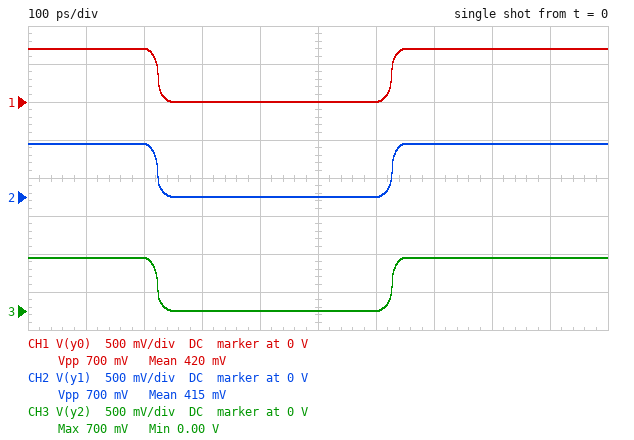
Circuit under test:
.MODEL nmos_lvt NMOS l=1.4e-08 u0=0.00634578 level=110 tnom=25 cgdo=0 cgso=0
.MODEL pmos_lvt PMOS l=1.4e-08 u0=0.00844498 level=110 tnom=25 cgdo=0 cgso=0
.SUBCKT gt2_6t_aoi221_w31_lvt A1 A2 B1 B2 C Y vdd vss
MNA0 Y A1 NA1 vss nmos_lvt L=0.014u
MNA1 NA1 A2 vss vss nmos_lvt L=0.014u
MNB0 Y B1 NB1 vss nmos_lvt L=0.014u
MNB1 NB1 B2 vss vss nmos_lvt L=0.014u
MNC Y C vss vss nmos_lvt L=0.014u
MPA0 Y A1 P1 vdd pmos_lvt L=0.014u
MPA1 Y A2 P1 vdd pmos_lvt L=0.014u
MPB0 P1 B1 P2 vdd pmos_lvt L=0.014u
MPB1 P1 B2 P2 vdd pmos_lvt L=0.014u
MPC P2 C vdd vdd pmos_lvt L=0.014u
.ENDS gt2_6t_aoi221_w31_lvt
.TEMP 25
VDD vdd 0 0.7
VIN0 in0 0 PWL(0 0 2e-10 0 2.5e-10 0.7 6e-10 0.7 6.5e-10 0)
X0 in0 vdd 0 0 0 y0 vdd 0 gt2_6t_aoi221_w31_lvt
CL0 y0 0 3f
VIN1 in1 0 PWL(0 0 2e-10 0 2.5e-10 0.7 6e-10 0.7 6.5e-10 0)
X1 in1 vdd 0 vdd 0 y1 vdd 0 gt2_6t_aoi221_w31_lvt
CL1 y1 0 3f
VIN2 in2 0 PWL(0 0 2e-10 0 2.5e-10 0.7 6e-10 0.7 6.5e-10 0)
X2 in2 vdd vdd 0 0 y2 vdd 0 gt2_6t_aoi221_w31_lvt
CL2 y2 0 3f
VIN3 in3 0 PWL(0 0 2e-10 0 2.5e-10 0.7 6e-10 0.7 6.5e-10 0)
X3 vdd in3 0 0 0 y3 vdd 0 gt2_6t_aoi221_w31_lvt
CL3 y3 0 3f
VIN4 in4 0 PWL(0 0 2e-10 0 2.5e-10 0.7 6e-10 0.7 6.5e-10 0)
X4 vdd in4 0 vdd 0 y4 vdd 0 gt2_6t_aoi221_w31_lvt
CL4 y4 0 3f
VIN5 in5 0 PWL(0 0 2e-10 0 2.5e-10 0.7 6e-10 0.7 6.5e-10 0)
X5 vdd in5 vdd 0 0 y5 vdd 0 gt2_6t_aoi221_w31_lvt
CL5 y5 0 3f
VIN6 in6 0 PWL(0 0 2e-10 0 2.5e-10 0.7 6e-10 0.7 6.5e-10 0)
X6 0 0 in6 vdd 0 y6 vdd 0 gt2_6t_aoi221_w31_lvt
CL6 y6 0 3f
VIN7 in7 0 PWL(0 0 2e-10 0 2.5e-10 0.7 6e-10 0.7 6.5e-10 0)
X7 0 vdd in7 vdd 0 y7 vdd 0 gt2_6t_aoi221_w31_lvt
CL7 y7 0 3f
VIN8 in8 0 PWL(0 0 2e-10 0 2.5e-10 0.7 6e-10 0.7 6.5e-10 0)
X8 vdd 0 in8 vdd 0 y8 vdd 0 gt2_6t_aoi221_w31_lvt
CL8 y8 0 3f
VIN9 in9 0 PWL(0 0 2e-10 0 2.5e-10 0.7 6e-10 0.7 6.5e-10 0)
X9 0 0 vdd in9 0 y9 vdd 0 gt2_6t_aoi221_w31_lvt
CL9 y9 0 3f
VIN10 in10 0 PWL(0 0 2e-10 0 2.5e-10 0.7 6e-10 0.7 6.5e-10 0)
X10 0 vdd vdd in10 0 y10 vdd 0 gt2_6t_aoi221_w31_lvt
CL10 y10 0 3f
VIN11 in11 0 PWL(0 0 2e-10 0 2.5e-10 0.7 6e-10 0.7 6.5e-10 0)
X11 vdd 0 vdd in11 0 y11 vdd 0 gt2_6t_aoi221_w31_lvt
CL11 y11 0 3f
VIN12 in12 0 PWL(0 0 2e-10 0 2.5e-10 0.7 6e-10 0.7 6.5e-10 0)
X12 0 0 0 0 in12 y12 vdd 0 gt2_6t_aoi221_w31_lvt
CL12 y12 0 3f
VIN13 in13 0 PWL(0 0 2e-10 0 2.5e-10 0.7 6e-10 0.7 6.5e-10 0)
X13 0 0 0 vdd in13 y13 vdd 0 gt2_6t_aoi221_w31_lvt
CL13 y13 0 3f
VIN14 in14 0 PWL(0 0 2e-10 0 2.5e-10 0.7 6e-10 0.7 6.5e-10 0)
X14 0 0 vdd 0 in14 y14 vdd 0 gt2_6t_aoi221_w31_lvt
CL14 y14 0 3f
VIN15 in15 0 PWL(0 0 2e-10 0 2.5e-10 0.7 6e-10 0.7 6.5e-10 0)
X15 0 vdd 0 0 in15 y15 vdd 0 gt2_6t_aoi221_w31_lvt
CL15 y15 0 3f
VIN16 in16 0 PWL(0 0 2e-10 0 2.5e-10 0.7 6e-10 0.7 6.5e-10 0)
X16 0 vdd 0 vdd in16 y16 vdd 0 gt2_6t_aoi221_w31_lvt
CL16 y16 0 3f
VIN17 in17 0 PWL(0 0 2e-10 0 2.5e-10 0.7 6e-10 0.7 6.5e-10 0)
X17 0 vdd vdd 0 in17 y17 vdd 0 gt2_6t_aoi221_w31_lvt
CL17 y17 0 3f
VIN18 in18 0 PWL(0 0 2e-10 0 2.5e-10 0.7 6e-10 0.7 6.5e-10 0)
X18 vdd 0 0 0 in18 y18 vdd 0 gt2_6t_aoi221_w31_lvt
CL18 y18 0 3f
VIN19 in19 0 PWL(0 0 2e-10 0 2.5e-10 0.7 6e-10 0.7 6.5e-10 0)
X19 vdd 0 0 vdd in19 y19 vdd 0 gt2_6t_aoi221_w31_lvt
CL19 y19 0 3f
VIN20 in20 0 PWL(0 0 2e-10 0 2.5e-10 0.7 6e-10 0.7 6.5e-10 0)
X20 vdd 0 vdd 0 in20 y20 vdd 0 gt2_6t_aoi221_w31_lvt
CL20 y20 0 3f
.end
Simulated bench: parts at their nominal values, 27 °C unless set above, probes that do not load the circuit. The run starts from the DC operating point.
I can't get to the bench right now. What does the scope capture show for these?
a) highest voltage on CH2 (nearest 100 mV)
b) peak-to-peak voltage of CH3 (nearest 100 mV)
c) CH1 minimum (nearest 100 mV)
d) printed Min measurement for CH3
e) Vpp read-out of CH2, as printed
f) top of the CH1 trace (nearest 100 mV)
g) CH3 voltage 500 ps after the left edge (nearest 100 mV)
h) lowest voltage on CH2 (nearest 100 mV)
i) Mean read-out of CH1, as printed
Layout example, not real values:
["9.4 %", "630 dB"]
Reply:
["700 mV", "700 mV", "0 V", "0.00 V", "700 mV", "700 mV", "0 V", "0 V", "420 mV"]
